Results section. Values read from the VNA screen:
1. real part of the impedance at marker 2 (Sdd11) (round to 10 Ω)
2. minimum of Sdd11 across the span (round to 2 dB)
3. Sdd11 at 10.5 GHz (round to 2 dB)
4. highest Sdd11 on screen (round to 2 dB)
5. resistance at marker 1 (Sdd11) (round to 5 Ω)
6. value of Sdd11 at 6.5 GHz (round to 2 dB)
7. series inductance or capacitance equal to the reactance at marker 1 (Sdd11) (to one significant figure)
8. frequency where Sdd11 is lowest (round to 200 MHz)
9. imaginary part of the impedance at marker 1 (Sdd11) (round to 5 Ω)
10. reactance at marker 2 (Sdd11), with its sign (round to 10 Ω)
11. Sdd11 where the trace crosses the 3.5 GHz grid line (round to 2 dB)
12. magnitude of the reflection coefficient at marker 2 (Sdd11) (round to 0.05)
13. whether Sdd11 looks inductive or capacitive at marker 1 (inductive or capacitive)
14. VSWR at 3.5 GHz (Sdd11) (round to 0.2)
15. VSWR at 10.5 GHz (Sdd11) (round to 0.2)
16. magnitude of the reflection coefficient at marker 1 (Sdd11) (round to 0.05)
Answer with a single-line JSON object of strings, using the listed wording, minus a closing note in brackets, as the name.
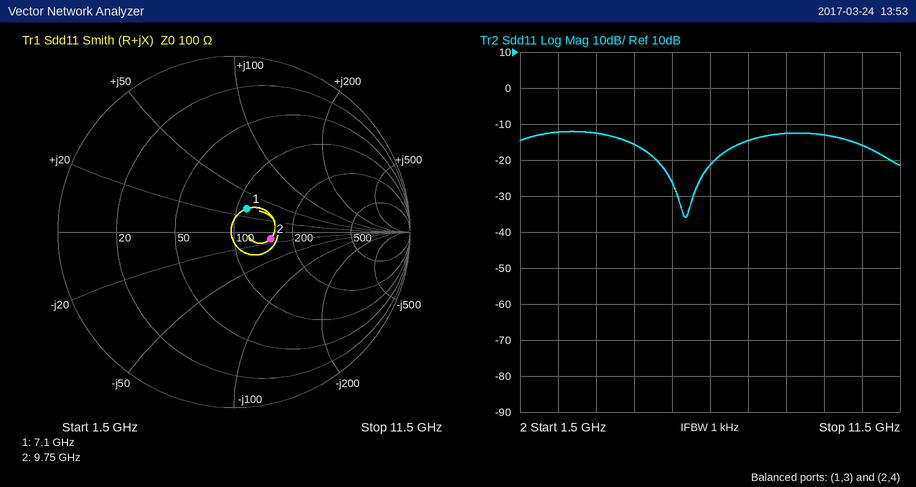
{"real part of the impedance at marker 2 (Sdd11)": "150 Ω", "minimum of Sdd11 across the span": "-36 dB", "Sdd11 at 10.5 GHz": "-16 dB", "highest Sdd11 on screen": "-12 dB", "resistance at marker 1 (Sdd11)": "110 Ω", "value of Sdd11 at 6.5 GHz": "-22 dB", "series inductance or capacitance equal to the reactance at marker 1 (Sdd11)": "700 pH", "frequency where Sdd11 is lowest": "5.8 GHz", "imaginary part of the impedance at marker 1 (Sdd11)": "+30 Ω", "reactance at marker 2 (Sdd11), with its sign": "-10 Ω", "Sdd11 where the trace crosses the 3.5 GHz grid line": "-12 dB", "magnitude of the reflection coefficient at marker 2 (Sdd11)": "0.20", "whether Sdd11 looks inductive or capacitive at marker 1": "inductive", "VSWR at 3.5 GHz (Sdd11)": "1.6", "VSWR at 10.5 GHz (Sdd11)": "1.4", "magnitude of the reflection coefficient at marker 1 (Sdd11)": "0.15"}
